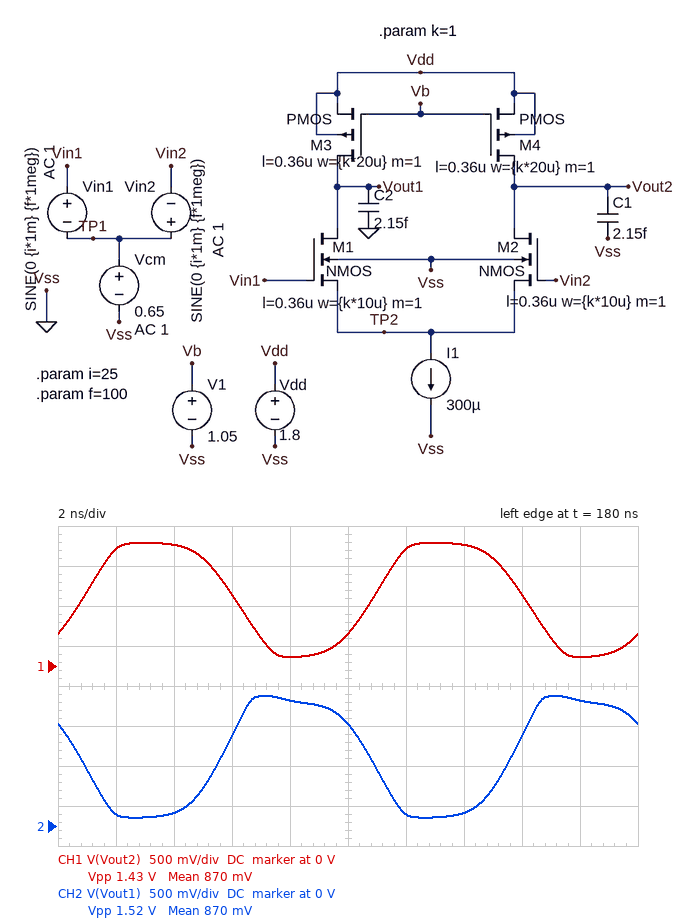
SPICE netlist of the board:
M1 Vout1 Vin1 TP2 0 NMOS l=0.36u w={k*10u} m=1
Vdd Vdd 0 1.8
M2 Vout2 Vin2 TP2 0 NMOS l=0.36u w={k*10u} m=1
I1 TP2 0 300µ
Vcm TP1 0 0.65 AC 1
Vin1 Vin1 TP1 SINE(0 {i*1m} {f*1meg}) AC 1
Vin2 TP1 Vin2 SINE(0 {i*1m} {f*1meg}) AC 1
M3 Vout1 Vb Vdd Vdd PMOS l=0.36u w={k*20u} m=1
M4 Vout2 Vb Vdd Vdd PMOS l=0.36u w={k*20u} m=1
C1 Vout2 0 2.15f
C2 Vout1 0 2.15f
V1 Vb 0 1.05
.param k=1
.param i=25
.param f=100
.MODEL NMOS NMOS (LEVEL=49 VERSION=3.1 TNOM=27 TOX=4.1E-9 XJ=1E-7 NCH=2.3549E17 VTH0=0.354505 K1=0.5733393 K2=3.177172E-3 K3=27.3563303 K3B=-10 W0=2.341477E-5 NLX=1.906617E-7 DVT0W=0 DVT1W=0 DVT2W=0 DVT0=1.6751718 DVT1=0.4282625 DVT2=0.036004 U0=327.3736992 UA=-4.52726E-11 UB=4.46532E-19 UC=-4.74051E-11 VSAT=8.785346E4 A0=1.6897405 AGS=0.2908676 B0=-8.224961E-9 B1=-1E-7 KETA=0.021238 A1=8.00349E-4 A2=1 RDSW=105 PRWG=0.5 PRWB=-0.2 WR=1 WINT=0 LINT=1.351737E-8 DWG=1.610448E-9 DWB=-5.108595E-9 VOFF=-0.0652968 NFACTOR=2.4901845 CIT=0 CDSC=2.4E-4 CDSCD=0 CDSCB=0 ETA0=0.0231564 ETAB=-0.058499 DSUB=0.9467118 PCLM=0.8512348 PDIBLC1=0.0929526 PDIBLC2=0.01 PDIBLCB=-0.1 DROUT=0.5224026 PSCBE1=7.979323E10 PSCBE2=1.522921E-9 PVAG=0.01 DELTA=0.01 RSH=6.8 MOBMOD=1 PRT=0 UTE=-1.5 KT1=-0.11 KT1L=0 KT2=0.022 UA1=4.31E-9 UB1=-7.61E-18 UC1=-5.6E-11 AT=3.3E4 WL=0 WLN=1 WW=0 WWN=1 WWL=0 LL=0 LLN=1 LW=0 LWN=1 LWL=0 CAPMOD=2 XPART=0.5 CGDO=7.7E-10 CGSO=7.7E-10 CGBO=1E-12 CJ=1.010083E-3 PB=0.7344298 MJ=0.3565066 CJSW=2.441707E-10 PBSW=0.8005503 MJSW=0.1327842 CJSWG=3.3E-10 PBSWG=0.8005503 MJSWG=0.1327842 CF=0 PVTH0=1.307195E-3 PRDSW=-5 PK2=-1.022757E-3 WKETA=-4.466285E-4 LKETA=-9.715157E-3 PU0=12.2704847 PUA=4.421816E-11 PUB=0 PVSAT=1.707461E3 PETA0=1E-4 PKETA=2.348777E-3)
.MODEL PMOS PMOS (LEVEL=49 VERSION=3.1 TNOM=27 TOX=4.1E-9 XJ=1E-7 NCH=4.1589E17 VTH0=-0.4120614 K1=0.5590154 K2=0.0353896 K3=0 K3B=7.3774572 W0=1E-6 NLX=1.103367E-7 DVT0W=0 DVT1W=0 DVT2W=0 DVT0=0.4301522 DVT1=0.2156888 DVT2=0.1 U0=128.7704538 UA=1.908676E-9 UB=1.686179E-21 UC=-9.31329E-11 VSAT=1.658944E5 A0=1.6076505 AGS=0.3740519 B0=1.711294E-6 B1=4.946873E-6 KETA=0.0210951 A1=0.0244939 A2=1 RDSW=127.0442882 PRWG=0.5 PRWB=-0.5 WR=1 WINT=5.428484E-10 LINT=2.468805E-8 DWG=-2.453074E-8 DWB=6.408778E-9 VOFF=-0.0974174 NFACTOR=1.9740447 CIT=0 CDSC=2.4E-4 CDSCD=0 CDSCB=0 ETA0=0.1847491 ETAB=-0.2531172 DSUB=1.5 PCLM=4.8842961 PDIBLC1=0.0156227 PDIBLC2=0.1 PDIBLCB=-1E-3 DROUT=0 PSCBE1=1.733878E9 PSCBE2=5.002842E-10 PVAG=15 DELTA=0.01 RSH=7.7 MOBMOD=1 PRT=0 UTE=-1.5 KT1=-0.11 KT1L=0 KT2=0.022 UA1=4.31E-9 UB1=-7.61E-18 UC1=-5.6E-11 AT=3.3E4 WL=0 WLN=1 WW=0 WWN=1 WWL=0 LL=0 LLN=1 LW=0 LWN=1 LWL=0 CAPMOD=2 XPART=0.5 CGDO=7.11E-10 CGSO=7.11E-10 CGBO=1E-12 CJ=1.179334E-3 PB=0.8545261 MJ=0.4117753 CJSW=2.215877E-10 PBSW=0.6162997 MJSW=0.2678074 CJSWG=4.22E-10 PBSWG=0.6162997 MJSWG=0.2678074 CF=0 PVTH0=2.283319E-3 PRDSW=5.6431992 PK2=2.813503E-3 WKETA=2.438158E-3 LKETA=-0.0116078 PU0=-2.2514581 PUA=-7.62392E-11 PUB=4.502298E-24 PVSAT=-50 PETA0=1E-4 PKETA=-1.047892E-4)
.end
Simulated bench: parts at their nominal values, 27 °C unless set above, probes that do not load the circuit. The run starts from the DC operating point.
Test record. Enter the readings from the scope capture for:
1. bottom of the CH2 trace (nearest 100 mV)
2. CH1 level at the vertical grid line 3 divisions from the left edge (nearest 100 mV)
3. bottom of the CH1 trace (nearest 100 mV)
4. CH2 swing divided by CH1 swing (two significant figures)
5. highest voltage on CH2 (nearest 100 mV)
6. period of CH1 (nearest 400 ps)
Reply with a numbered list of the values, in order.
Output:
1. 100 mV
2. 900 mV
3. 100 mV
4. 1.1
5. 1.6 V
6. 10.0 ns
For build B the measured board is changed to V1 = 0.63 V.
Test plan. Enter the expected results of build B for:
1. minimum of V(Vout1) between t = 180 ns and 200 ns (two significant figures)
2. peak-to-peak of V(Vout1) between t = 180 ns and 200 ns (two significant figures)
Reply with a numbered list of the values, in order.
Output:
1. 1.7 V
2. 32 mV
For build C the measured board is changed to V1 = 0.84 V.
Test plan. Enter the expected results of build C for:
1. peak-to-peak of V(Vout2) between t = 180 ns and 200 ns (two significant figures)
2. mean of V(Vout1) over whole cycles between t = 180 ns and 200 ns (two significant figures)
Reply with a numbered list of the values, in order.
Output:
1. 49 mV
2. 1.7 V
